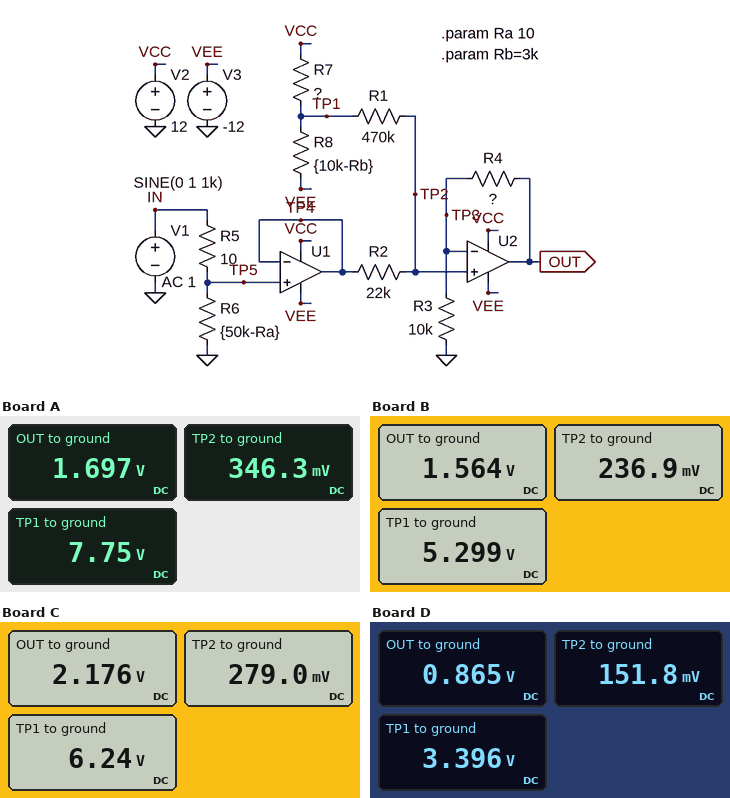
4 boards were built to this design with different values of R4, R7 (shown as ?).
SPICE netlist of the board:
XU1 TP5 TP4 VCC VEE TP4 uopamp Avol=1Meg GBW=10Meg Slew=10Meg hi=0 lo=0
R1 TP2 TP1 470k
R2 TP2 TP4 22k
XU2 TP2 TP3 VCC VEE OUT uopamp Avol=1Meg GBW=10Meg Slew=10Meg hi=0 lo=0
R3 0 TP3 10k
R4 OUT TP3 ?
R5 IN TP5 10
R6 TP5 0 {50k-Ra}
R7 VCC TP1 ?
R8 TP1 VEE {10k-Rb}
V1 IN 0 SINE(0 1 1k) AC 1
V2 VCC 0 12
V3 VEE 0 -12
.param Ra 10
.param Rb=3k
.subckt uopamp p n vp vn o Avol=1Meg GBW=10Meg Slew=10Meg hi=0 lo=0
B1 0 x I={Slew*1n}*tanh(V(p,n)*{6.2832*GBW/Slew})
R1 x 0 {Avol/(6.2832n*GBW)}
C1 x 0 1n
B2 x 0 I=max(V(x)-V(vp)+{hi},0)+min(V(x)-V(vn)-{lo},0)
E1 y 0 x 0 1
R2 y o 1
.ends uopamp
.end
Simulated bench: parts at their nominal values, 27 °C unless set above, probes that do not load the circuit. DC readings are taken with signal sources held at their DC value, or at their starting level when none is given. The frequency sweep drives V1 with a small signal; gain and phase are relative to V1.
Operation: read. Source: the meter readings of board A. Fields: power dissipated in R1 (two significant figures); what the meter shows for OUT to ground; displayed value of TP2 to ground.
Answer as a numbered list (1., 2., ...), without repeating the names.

1. 120 µW
2. 1.697 V
3. 346.3 mV
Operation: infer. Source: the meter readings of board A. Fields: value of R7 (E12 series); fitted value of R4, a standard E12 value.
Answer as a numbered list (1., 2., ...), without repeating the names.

1. 1.5 kΩ
2. 39 kΩ
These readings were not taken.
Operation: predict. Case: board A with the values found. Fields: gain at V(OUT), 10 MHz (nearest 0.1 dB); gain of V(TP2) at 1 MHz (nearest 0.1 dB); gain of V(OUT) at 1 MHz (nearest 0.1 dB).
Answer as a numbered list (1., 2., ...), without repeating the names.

1. -3.6 dB
2. -0.4 dB
3. 12.4 dB
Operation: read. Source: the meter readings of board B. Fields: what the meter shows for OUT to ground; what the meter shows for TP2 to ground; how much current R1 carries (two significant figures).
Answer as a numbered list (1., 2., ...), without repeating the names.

1. 1.564 V
2. 236.9 mV
3. 11 µA
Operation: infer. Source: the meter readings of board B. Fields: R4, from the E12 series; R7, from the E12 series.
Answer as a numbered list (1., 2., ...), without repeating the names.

1. 56 kΩ
2. 2.7 kΩ
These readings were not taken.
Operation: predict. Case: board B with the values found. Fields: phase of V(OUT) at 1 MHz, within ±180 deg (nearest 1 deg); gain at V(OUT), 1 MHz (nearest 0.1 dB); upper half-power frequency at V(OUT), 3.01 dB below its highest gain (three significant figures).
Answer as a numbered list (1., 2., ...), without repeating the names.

1. -39 deg
2. 14.4 dB
3. 1.48 MHz
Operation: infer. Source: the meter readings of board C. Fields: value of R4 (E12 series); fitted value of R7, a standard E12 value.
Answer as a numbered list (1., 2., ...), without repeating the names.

1. 68 kΩ
2. 2.2 kΩ
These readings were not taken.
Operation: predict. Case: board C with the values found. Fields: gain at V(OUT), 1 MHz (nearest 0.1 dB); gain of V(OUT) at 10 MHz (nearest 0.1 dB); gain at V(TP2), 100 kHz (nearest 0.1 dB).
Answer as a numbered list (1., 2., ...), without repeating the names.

1. 15.3 dB
2. -3.5 dB
3. -0.4 dB
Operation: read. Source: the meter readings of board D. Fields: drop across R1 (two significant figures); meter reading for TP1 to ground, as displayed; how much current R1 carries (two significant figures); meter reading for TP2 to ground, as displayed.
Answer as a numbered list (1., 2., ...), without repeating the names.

1. 3.2 V
2. 3.396 V
3. 6.9 µA
4. 151.8 mV
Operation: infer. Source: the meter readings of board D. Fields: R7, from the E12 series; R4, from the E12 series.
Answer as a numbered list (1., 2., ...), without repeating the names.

1. 3.9 kΩ
2. 47 kΩ
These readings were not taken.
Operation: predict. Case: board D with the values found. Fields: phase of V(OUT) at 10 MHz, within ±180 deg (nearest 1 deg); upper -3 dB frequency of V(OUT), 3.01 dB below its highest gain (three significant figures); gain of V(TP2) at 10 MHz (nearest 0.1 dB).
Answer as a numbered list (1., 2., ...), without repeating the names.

1. -125 deg
2. 1.70 MHz
3. -3.4 dB
